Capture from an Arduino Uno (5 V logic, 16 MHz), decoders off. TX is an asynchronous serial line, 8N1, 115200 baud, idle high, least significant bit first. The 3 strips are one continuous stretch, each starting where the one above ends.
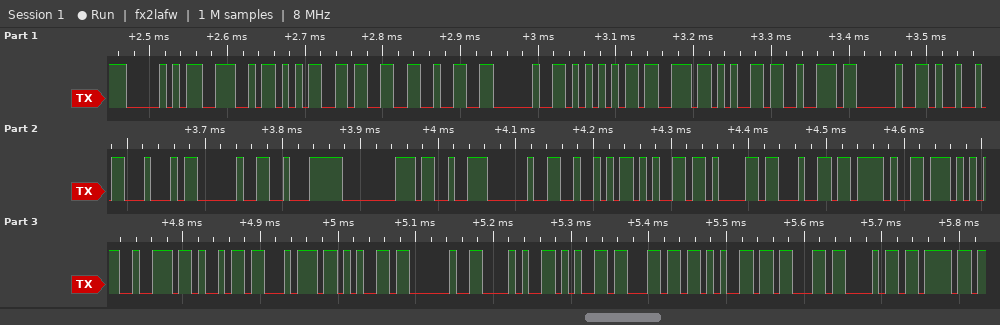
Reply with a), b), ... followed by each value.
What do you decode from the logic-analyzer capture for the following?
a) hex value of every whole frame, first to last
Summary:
a) 50 4E 35 33 32 20 55 73 65 72 20 49 44 20 E2 80 93 20 52 65 61 64 2F 57 72 69 74 65 20 28 65 6C 65 63 68 6F
